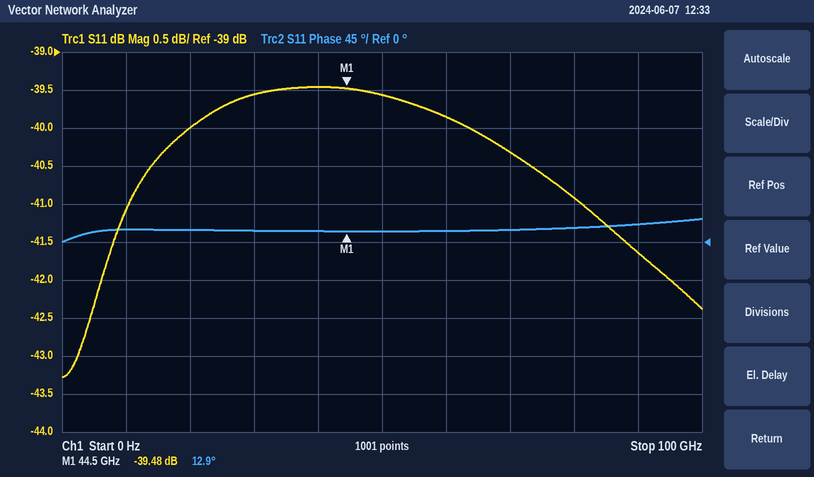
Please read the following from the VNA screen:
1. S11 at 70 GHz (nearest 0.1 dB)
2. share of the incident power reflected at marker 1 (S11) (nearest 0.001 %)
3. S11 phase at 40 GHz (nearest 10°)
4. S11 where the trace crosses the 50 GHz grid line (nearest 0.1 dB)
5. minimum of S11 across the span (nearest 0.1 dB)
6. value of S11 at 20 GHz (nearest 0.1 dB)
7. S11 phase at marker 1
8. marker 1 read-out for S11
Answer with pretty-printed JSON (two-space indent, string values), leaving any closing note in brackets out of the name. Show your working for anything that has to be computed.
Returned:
{
  "S11 at 70 GHz": "-40.3 dB",
  "share of the incident power reflected at marker 1 (S11)": "10^(-39.48/10) ≈ 0.011 %",
  "S11 phase at 40 GHz": "10°",
  "S11 where the trace crosses the 50 GHz grid line": "-39.6 dB",
  "minimum of S11 across the span": "-43.3 dB",
  "value of S11 at 20 GHz": "-40.0 dB",
  "S11 phase at marker 1": "12.9°",
  "marker 1 read-out for S11": "-39.48 dB"
}
